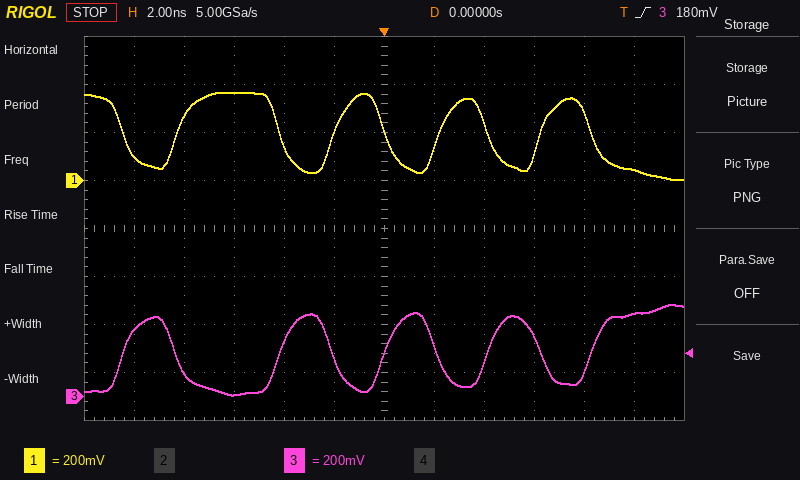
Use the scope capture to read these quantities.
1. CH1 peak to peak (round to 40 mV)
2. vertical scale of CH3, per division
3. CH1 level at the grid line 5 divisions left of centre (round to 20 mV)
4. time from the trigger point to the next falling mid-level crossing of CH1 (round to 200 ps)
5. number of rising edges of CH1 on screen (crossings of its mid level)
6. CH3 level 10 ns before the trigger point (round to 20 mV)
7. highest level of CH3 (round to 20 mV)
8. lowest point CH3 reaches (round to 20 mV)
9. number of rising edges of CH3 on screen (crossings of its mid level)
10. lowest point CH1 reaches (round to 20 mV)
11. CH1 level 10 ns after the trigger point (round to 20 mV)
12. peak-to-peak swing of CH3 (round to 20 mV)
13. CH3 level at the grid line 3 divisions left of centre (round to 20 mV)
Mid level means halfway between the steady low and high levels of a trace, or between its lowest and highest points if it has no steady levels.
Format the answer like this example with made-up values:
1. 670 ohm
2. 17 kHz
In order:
1. 360 mV
2. 200 mV
3. 100 mV
4. 4.2 ns
5. 4
6. 280 mV
7. 380 mV
8. 0 mV
9. 5
10. 0 mV
11. 40 mV
12. 380 mV
13. 0 mV
